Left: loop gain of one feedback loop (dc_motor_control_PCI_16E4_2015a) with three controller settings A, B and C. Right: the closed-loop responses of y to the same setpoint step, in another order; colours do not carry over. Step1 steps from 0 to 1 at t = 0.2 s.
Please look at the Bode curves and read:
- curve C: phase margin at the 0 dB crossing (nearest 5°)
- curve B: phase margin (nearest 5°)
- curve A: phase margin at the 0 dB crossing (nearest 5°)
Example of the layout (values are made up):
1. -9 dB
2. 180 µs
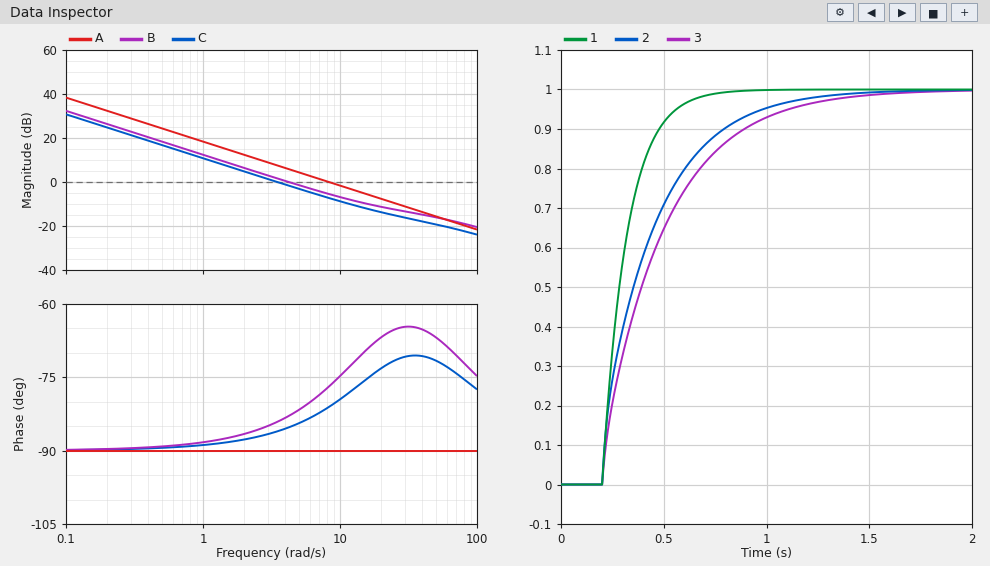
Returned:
1. 95°
2. 95°
3. 90°
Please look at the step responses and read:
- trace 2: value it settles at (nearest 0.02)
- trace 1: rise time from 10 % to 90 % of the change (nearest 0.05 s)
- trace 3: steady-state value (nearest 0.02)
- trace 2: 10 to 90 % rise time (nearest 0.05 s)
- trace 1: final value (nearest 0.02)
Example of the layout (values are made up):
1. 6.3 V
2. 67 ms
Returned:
1. 1.00
2. 0.25 s
3. 1.00
4. 0.60 s
5. 1.00
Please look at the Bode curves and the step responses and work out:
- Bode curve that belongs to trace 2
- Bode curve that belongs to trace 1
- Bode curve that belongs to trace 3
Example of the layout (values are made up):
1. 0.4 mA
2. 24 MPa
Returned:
1. B
2. A
3. C
